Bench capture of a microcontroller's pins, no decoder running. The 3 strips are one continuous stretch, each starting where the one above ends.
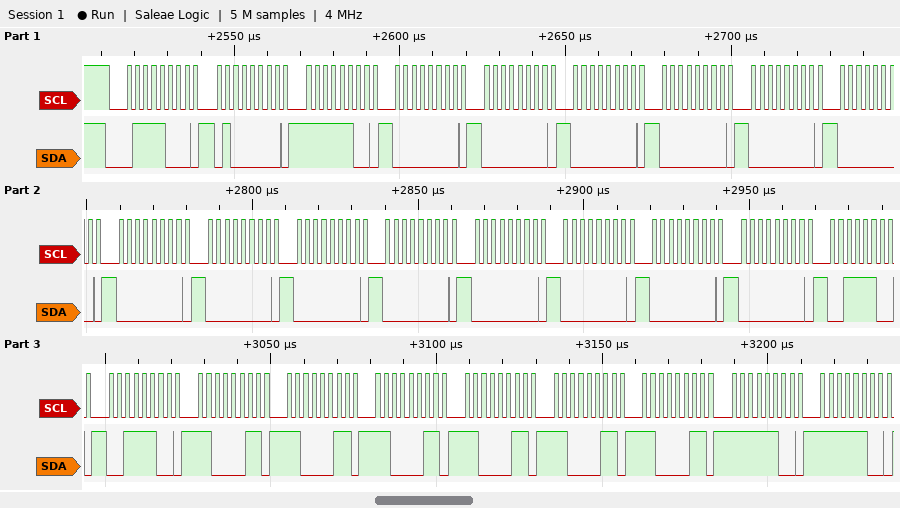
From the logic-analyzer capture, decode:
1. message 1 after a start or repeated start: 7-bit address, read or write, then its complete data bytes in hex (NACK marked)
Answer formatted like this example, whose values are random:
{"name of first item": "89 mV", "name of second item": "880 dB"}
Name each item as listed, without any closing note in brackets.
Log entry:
{"message 1 after a start or repeated start: 7-bit address, read or write, then its complete data bytes in hex": "0x3C write: 40 FC 00 00 00 00 00 00 00 00 00 00 00 00 00 00 3C 3C C3 C3 C3 C3 C3 C3 FC FC"}
